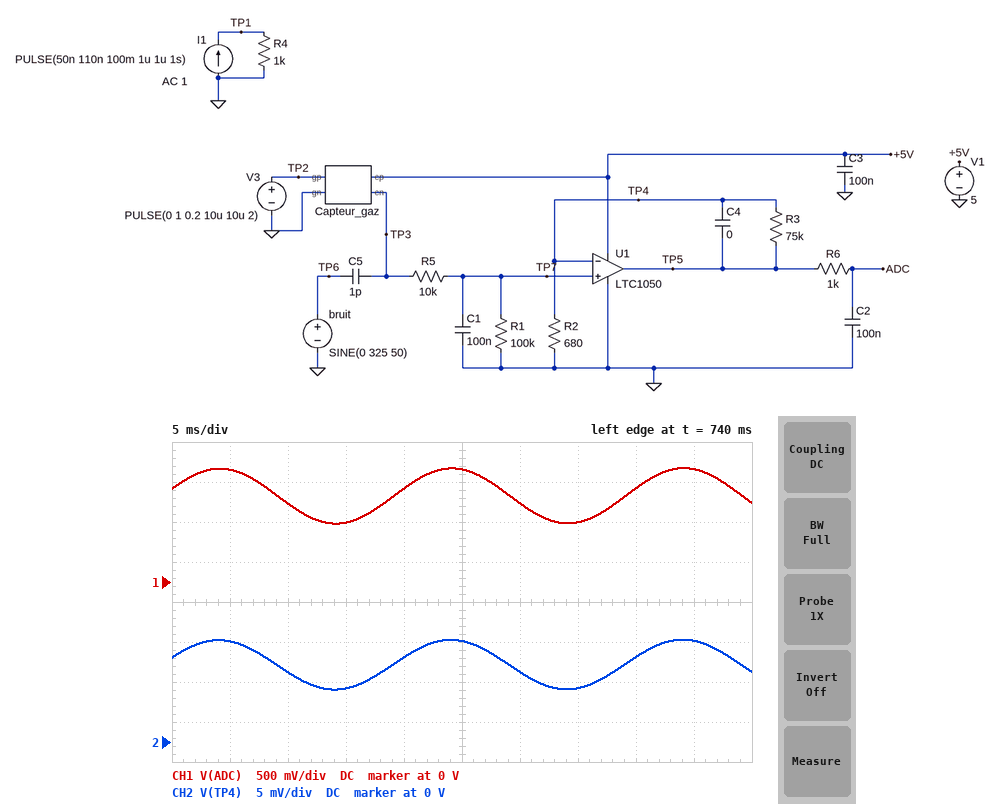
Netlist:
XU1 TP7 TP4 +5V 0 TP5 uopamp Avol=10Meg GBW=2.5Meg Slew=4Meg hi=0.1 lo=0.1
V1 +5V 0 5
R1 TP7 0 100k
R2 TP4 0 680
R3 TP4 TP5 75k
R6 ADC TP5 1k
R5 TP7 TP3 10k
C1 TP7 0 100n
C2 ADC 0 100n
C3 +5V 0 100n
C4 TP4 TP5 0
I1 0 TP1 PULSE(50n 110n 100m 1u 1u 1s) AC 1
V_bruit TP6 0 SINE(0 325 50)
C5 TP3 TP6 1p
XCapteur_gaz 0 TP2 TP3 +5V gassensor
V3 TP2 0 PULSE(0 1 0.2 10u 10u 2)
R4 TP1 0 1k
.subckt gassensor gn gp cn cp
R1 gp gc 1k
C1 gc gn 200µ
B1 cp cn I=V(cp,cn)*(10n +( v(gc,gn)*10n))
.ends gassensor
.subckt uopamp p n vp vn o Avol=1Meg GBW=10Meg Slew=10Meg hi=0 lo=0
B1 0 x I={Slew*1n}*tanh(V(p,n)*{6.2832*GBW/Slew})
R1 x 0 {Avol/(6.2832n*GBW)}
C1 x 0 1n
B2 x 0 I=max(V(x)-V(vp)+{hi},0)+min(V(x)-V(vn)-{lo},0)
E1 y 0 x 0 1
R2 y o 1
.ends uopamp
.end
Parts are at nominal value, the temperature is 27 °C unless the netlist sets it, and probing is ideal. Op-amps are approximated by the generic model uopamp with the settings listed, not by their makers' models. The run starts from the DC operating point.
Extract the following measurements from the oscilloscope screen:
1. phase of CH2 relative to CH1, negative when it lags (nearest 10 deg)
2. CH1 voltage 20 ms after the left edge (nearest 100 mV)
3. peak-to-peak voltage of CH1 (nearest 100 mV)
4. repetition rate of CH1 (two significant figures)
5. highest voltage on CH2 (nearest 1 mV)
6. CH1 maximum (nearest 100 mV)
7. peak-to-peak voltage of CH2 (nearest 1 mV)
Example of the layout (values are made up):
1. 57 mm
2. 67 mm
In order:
1. 0 deg
2. 1.2 V
3. 700 mV
4. 50 Hz
5. 13 mV
6. 1.4 V
7. 6 mV
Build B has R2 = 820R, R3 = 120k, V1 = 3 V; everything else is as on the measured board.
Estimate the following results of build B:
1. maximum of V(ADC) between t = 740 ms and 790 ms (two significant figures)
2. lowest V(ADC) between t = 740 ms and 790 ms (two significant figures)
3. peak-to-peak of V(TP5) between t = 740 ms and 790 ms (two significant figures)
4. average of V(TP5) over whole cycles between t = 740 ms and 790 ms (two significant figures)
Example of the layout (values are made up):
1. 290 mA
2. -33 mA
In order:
1. 1.3 V
2. 400 mV
3. 920 mV
4. 850 mV
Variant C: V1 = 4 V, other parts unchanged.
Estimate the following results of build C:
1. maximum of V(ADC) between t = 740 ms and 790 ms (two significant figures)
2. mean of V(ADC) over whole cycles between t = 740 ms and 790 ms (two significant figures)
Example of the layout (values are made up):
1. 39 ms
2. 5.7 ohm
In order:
1. 1.2 V
2. 860 mV
